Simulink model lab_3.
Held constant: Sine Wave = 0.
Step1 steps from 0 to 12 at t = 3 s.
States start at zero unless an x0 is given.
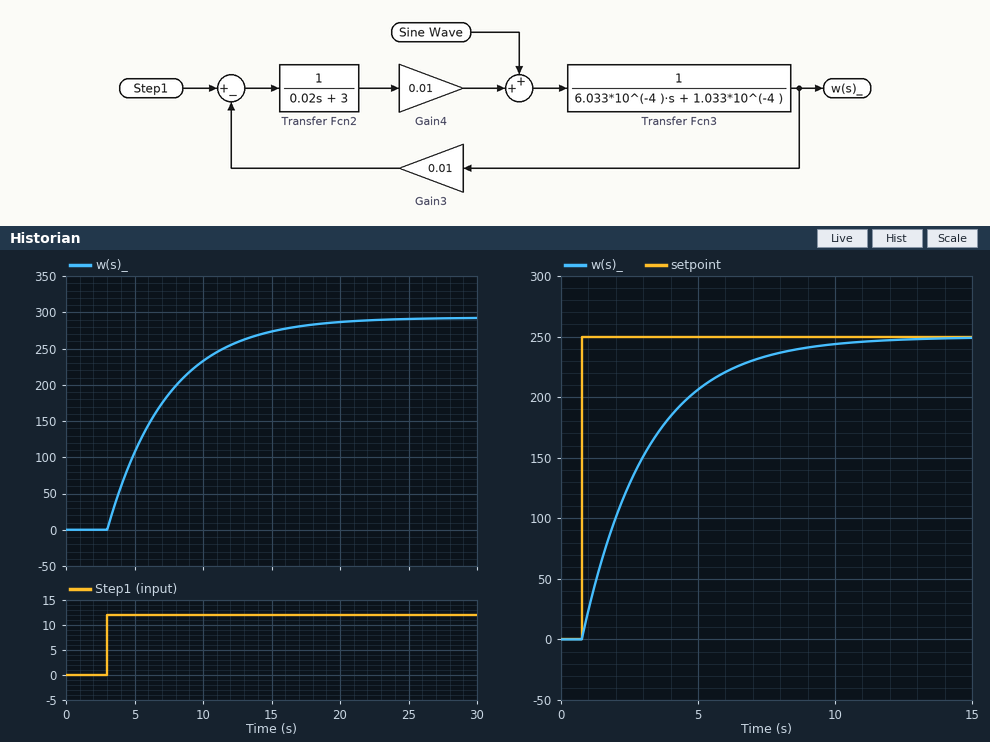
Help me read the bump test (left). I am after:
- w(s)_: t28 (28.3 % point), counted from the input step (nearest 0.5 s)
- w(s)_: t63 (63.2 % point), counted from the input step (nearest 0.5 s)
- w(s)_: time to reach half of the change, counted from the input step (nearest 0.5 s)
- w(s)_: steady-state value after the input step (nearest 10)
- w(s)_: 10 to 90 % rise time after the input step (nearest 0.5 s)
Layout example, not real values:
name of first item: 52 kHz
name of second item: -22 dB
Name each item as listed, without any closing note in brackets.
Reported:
w(s)_: t28 (28.3 % point), counted from the input step: 1.5 s
w(s)_: t63 (63.2 % point), counted from the input step: 4.5 s
w(s)_: time to reach half of the change, counted from the input step: 3.0 s
w(s)_: steady-state value after the input step: 290
w(s)_: 10 to 90 % rise time after the input step: 9.5 s
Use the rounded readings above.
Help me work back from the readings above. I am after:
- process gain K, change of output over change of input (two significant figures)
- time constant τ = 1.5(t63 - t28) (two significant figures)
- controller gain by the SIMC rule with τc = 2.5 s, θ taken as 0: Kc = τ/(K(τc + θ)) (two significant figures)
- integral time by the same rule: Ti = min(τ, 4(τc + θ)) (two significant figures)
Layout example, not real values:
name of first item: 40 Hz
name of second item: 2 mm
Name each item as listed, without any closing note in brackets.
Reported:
process gain K, change of output over change of input: 24
time constant τ = 1.5(t63 - t28): 4.5 s
controller gain by the SIMC rule with τc = 2.5 s, θ taken as 0: Kc = τ/(K(τc + θ)): 0.075
integral time by the same rule: Ti = min(τ, 4(τc + θ)): 4.5 s
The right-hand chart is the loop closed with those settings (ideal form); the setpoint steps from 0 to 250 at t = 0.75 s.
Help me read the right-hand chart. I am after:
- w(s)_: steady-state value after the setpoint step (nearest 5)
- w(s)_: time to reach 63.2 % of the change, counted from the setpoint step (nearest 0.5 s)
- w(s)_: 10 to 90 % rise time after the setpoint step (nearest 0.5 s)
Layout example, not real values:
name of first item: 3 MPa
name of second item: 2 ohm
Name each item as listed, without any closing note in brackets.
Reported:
w(s)_: steady-state value after the setpoint step: 250
w(s)_: time to reach 63.2 % of the change, counted from the setpoint step: 2.5 s
w(s)_: 10 to 90 % rise time after the setpoint step: 5.5 s
